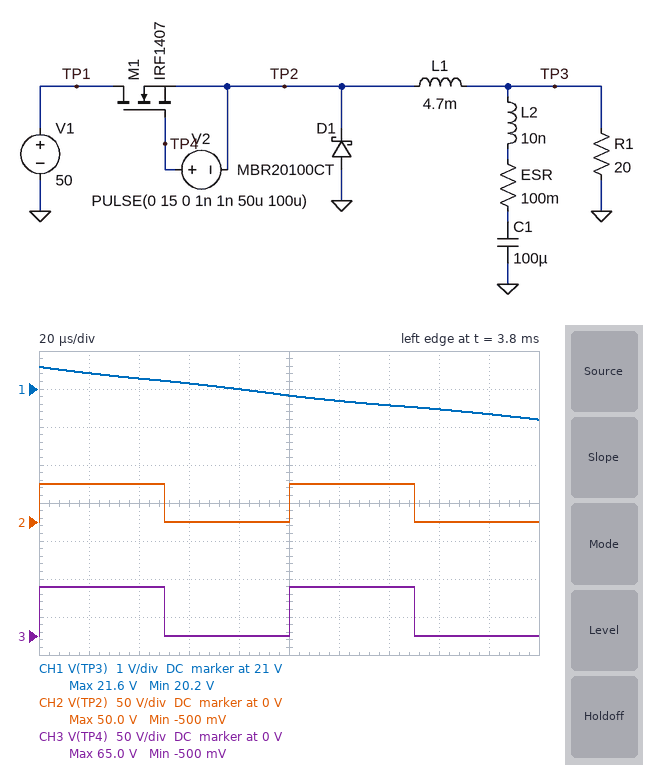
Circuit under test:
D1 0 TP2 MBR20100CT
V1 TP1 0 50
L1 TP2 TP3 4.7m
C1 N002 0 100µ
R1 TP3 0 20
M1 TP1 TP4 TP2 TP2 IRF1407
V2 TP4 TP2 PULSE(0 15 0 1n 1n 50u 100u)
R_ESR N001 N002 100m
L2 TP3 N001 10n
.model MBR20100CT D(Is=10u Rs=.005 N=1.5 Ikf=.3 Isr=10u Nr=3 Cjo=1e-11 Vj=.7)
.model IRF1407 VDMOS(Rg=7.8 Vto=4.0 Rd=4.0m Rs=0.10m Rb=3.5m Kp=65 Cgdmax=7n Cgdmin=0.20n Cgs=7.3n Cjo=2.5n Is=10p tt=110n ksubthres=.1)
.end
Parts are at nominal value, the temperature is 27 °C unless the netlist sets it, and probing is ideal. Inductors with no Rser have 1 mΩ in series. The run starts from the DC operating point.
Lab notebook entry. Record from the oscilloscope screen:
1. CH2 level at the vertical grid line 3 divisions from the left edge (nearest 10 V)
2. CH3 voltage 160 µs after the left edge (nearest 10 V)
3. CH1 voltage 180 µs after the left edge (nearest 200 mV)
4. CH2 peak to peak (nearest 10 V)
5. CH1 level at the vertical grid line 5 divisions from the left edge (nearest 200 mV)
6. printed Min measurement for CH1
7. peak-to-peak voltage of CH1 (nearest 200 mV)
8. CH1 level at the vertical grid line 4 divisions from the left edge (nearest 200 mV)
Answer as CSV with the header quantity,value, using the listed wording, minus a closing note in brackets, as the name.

quantity,value
CH2 level at the vertical grid line 3 divisions from the left edge,0 V
CH3 voltage 160 µs after the left edge,0 V
CH1 voltage 180 µs after the left edge,20.4 V
CH2 peak to peak,50 V
CH1 level at the vertical grid line 5 divisions from the left edge,20.8 V
printed Min measurement for CH1,20.2 V
peak-to-peak voltage of CH1,1.4 V
CH1 level at the vertical grid line 4 divisions from the left edge,21.0 V
